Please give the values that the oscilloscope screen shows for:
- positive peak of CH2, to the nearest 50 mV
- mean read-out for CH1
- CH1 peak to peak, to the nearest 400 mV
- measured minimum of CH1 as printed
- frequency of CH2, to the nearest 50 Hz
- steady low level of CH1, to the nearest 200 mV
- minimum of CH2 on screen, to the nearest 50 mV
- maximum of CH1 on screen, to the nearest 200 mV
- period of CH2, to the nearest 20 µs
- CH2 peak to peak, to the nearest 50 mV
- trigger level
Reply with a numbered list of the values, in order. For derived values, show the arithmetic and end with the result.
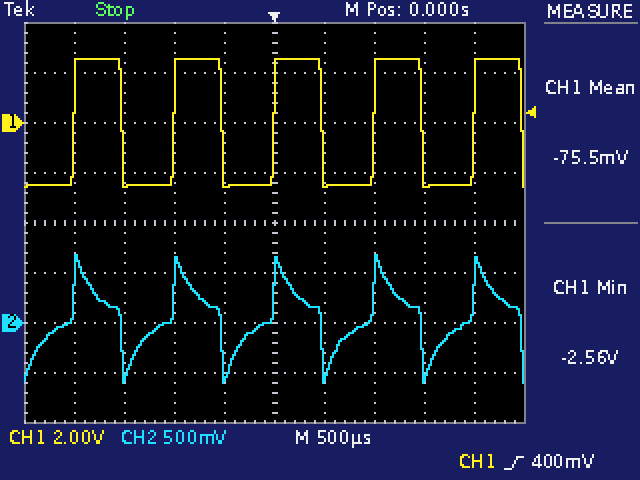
1. 700 mV
2. -75.5 mV
3. 5.2 V
4. -2.56 V
5. 1 / 1.00 ms ≈ 1.00 kHz
6. -2.4 V
7. -600 mV
8. 2.6 V
9. 1.00 ms
10. 700 mV − (-600 mV) = 1.30 V
11. 400 mV
